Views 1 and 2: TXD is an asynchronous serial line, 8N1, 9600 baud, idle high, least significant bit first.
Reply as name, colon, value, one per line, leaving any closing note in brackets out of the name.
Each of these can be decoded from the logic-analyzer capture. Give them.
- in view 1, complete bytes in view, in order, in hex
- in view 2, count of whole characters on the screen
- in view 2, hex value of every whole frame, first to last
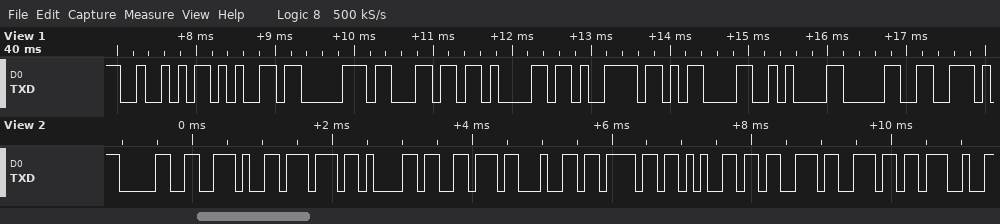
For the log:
in view 1, complete bytes in view, in order, in hex: 0x52 0x65 0x70 0x6C 0x61 0x79 0x0D 0x0A 0x30
in view 2, count of whole characters on the screen: 11
in view 2, hex value of every whole frame, first to last: 30 2E 77 61 76 64 6F 65 73 6E 27
